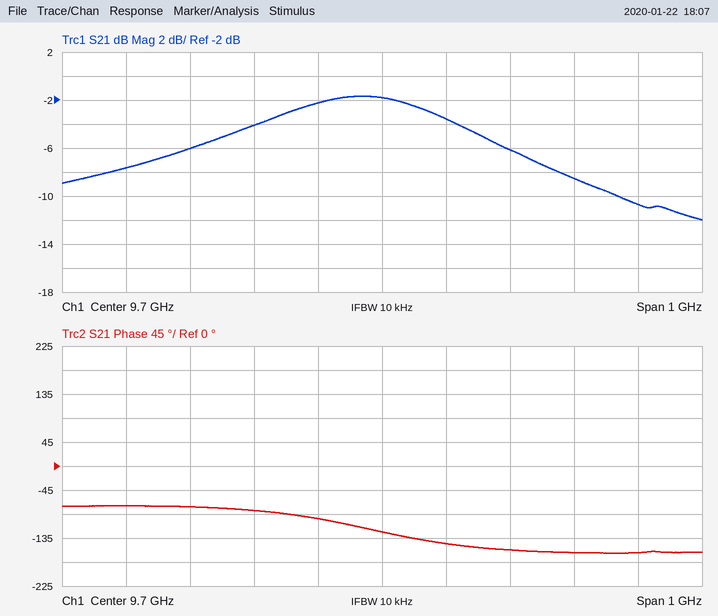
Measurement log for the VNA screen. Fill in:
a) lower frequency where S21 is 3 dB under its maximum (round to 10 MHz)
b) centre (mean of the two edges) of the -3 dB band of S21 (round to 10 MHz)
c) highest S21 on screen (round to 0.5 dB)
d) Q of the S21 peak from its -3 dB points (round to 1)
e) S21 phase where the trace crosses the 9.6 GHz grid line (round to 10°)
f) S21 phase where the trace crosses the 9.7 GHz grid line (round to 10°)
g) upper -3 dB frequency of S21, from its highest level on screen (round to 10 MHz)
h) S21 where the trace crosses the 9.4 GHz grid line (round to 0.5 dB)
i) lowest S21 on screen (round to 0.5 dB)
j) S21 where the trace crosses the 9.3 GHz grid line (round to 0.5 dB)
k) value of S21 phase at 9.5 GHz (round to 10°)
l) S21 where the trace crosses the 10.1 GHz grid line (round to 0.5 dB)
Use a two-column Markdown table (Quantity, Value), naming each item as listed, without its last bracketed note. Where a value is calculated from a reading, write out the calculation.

| Quantity | Value |
|---|---|
| lower frequency where S21 is 3 dB under its maximum | 9.47 GHz |
| centre (mean of the two edges) of the -3 dB band of S21 | 9.66 GHz |
| highest S21 on screen | -1.5 dB |
| Q of the S21 peak from its -3 dB points | 9.655 GHz / 370 MHz ≈ 26 |
| S21 phase where the trace crosses the 9.6 GHz grid line | -100° |
| S21 phase where the trace crosses the 9.7 GHz grid line | -120° |
| upper -3 dB frequency of S21, from its highest level on screen | 9.84 GHz |
| S21 where the trace crosses the 9.4 GHz grid line | -6.0 dB |
| lowest S21 on screen | -12.0 dB |
| S21 where the trace crosses the 9.3 GHz grid line | -7.5 dB |
| value of S21 phase at 9.5 GHz | -80° |
| S21 where the trace crosses the 10.1 GHz grid line | -10.5 dB |
